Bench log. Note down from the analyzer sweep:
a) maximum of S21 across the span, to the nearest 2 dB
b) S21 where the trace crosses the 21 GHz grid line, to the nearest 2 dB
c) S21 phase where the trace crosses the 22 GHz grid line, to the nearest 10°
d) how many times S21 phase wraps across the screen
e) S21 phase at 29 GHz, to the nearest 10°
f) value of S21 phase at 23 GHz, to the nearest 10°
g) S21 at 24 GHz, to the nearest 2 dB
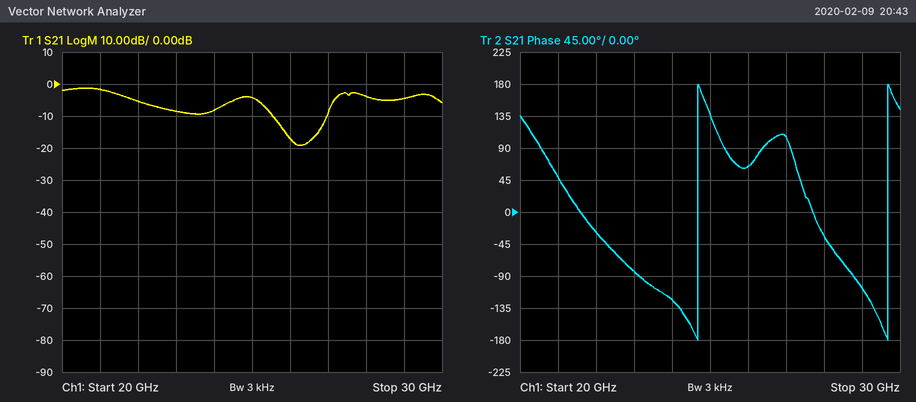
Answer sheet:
-2 dB
-2 dB
-30°
2
-110°
-80°
-8 dB
